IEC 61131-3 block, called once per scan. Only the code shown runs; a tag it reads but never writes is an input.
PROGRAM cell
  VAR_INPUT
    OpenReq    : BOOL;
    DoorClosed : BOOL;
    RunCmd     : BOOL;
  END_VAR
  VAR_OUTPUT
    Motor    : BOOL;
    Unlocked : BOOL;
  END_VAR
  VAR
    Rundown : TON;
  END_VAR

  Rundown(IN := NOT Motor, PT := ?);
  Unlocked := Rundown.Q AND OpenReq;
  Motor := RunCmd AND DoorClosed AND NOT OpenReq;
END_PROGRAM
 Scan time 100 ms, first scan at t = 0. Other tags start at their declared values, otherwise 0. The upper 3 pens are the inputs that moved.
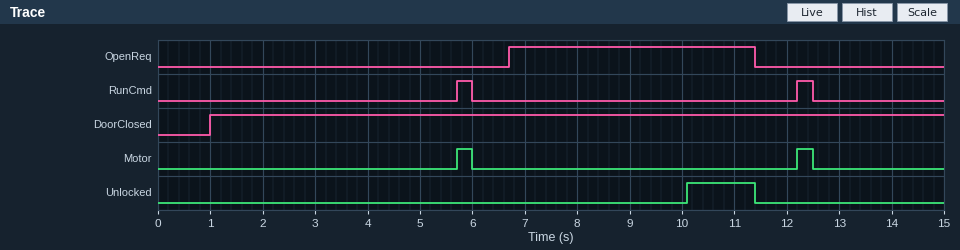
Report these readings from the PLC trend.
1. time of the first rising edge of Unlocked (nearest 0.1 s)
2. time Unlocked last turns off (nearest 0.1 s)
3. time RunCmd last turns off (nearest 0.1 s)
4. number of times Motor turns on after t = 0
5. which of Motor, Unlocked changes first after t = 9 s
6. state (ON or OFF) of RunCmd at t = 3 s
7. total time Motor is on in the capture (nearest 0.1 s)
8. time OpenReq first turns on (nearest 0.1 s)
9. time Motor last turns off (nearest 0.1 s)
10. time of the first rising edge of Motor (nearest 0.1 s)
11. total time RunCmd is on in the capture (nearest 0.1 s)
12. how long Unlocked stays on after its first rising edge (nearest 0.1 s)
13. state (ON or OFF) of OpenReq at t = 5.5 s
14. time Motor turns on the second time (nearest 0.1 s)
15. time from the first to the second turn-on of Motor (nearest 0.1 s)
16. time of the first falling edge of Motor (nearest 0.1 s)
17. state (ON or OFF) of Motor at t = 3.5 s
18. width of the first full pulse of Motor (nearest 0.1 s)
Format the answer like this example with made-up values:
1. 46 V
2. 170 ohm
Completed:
1. 10.1 s
2. 11.4 s
3. 12.5 s
4. 2
5. Unlocked
6. OFF
7. 0.6 s
8. 6.7 s
9. 12.5 s
10. 5.7 s
11. 0.6 s
12. 1.3 s
13. OFF
14. 12.2 s
15. 6.5 s
16. 6.0 s
17. OFF
18. 0.3 s
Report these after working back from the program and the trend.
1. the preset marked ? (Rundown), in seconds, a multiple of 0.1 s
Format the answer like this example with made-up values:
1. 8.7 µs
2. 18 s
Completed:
1. 4.0 s
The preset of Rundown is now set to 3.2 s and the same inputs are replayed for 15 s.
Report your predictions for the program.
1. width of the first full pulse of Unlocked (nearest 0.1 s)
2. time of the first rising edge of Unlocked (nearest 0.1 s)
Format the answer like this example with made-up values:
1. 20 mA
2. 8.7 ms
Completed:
1. 2.1 s
2. 9.3 s
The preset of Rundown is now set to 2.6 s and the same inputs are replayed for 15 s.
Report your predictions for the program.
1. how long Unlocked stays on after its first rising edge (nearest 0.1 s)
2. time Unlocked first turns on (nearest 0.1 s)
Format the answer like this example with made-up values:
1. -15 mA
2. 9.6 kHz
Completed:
1. 2.7 s
2. 8.7 s
